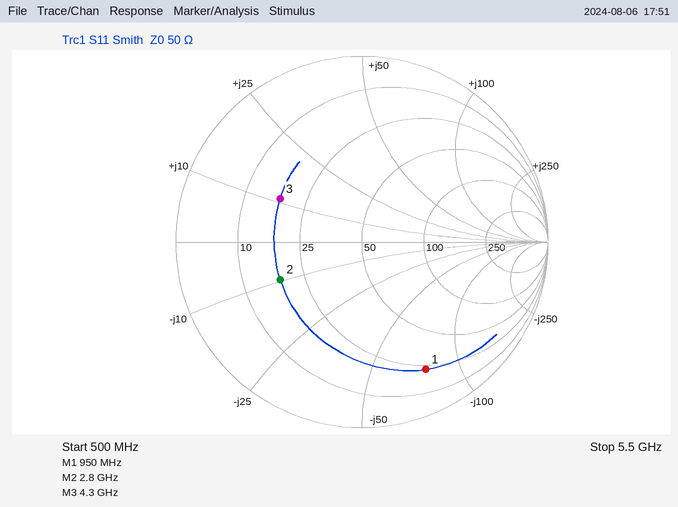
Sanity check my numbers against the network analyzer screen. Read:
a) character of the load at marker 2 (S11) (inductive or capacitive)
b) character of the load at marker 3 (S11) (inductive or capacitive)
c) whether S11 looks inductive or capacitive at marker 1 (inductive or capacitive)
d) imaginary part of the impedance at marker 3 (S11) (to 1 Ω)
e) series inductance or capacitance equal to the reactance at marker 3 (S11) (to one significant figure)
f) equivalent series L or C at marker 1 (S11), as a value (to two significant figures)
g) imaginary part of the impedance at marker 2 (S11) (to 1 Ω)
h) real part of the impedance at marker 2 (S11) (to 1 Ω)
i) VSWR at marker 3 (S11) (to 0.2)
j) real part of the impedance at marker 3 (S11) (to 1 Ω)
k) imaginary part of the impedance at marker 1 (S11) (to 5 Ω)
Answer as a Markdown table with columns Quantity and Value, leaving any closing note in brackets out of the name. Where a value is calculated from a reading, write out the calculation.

| Quantity | Value |
|---|---|
| character of the load at marker 2 (S11) | capacitive |
| character of the load at marker 3 (S11) | inductive |
| whether S11 looks inductive or capacitive at marker 1 | capacitive |
| imaginary part of the impedance at marker 3 (S11) | +11 Ω |
| series inductance or capacitance equal to the reactance at marker 3 (S11) | L = 11 Ω/(2π × 4.3 GHz) ≈ 407 pH, so 400 pH to one significant figure |
| equivalent series L or C at marker 1 (S11), as a value | C = 1/(2π × 950 MHz × 75 Ω) ≈ 2.2 pF |
| imaginary part of the impedance at marker 2 (S11) | -10 Ω |
| real part of the impedance at marker 2 (S11) | 18 Ω |
| VSWR at marker 3 (S11) | 3.0 |
| real part of the impedance at marker 3 (S11) | 18 Ω |
| imaginary part of the impedance at marker 1 (S11) | -75 Ω |
